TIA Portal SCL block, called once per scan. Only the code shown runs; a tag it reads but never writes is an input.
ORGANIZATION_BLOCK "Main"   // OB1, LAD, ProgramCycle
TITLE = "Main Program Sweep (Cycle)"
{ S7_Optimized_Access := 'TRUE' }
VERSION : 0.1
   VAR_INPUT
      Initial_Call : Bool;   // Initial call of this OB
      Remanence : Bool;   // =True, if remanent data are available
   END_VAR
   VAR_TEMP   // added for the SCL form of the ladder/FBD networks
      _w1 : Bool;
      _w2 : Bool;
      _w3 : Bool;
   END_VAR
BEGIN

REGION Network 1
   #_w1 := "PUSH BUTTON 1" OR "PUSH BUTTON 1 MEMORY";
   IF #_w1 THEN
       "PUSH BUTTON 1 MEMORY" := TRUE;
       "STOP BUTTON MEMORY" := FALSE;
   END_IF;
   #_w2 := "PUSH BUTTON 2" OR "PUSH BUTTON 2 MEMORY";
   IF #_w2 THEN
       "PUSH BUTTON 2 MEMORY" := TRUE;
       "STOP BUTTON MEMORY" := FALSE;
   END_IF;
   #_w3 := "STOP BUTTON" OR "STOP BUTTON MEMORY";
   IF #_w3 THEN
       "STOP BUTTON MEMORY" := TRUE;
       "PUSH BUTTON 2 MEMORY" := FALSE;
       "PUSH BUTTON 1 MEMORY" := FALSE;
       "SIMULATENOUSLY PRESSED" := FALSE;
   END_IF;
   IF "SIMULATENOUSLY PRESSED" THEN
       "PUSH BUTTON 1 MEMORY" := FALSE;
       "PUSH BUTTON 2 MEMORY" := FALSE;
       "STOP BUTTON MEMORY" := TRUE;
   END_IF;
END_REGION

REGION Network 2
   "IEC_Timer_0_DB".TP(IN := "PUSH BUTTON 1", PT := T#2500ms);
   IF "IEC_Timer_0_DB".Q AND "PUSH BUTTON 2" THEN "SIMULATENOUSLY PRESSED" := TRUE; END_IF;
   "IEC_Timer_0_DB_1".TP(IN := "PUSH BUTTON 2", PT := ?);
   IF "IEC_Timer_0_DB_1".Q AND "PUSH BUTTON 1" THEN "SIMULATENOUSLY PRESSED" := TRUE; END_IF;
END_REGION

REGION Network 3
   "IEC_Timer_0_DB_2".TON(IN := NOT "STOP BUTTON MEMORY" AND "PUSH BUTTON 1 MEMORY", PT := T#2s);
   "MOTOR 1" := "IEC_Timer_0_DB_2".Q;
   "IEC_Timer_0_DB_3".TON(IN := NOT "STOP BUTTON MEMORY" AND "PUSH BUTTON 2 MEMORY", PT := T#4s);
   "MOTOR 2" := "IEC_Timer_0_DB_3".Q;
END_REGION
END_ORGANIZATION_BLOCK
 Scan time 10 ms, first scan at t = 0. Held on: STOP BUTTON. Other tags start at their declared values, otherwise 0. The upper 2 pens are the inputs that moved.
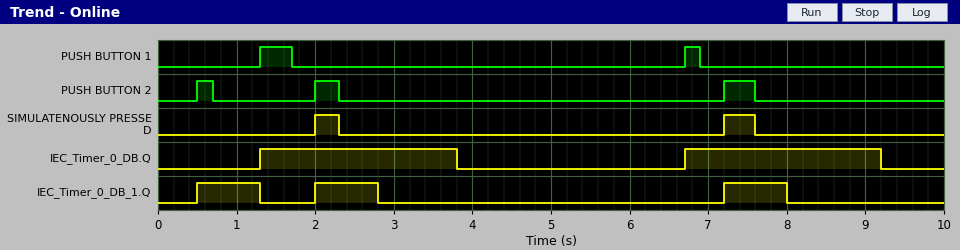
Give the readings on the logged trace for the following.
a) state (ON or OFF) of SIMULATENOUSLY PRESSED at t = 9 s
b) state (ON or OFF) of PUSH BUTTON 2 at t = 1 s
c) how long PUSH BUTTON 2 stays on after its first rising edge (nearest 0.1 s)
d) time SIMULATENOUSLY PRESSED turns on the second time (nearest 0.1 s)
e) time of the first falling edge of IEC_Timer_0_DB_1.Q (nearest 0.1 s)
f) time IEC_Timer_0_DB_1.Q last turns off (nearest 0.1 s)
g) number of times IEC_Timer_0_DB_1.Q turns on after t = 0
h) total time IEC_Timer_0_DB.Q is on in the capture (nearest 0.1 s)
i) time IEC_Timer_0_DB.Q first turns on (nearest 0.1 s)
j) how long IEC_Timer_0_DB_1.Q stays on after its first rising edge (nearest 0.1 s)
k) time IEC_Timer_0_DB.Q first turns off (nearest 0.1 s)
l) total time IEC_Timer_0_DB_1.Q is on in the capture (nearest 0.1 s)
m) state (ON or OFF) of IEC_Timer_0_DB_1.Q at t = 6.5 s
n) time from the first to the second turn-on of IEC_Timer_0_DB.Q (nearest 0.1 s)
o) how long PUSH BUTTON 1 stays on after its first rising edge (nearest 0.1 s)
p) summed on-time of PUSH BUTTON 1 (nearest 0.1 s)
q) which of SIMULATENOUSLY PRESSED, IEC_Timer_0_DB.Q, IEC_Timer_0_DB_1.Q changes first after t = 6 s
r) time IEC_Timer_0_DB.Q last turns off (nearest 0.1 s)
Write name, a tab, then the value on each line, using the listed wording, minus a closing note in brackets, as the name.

state (ON or OFF) of SIMULATENOUSLY PRESSED at t = 9 s	OFF
state (ON or OFF) of PUSH BUTTON 2 at t = 1 s	OFF
how long PUSH BUTTON 2 stays on after its first rising edge	0.2 s
time SIMULATENOUSLY PRESSED turns on the second time	7.2 s
time of the first falling edge of IEC_Timer_0_DB_1.Q	1.3 s
time IEC_Timer_0_DB_1.Q last turns off	8.0 s
number of times IEC_Timer_0_DB_1.Q turns on after t = 0	3
total time IEC_Timer_0_DB.Q is on in the capture	5.0 s
time IEC_Timer_0_DB.Q first turns on	1.3 s
how long IEC_Timer_0_DB_1.Q stays on after its first rising edge	0.8 s
time IEC_Timer_0_DB.Q first turns off	3.8 s
total time IEC_Timer_0_DB_1.Q is on in the capture	2.4 s
state (ON or OFF) of IEC_Timer_0_DB_1.Q at t = 6.5 s	OFF
time from the first to the second turn-on of IEC_Timer_0_DB.Q	5.4 s
how long PUSH BUTTON 1 stays on after its first rising edge	0.4 s
summed on-time of PUSH BUTTON 1	0.6 s
which of SIMULATENOUSLY PRESSED, IEC_Timer_0_DB.Q, IEC_Timer_0_DB_1.Q changes first after t = 6 s	IEC_Timer_0_DB.Q
time IEC_Timer_0_DB.Q last turns off	9.2 s
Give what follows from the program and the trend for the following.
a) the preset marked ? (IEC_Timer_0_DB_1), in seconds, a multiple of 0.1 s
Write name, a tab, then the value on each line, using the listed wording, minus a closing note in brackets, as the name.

the preset marked ? (IEC_Timer_0_DB_1), in seconds, a multiple of 0.1 s	0.8 s
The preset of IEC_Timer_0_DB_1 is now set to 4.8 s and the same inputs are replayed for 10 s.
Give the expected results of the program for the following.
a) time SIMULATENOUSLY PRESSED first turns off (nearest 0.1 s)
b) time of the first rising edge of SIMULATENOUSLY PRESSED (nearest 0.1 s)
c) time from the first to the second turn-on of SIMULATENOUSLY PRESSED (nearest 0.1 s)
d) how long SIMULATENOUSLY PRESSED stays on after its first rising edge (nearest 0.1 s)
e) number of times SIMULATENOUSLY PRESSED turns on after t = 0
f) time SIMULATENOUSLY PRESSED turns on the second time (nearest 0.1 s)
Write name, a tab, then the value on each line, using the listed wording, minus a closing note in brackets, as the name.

time SIMULATENOUSLY PRESSED first turns off	1.7 s
time of the first rising edge of SIMULATENOUSLY PRESSED	1.3 s
time from the first to the second turn-on of SIMULATENOUSLY PRESSED	0.7 s
how long SIMULATENOUSLY PRESSED stays on after its first rising edge	0.4 s
number of times SIMULATENOUSLY PRESSED turns on after t = 0	3
time SIMULATENOUSLY PRESSED turns on the second time	2.0 s
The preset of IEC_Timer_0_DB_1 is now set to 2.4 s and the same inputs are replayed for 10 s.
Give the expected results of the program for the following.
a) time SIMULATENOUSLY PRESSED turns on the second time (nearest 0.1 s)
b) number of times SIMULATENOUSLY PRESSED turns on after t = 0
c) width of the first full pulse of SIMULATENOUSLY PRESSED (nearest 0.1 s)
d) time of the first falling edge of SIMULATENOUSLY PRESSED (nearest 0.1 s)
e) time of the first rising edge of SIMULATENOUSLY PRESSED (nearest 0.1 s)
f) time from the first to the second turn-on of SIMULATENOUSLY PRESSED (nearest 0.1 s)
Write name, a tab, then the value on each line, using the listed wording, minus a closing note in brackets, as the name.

time SIMULATENOUSLY PRESSED turns on the second time	2.0 s
number of times SIMULATENOUSLY PRESSED turns on after t = 0	3
width of the first full pulse of SIMULATENOUSLY PRESSED	0.4 s
time of the first falling edge of SIMULATENOUSLY PRESSED	1.7 s
time of the first rising edge of SIMULATENOUSLY PRESSED	1.3 s
time from the first to the second turn-on of SIMULATENOUSLY PRESSED	0.7 s
